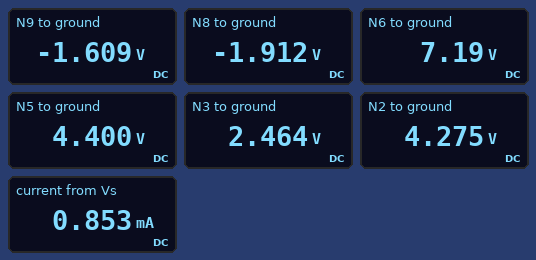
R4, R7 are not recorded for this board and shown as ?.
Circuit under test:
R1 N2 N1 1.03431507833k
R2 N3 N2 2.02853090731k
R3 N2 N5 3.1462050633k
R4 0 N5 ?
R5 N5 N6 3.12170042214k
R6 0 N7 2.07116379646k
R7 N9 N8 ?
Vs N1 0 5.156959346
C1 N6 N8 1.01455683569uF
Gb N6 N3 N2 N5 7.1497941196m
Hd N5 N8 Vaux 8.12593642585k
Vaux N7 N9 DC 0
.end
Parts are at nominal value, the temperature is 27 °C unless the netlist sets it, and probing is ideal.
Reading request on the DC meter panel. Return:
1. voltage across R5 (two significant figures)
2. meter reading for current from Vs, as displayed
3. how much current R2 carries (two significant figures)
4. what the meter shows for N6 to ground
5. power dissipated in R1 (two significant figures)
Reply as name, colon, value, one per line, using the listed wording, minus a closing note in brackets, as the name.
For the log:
voltage across R5: 2.8 V
meter reading for current from Vs, as displayed: 0.853 mA
how much current R2 carries: 890 µA
what the meter shows for N6 to ground: 7.19 V
power dissipated in R1: 750 µW
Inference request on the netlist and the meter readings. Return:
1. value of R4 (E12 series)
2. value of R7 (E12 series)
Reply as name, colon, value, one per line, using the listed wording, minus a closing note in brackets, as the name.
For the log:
value of R4: 2.7 kΩ
value of R7: 390 Ω
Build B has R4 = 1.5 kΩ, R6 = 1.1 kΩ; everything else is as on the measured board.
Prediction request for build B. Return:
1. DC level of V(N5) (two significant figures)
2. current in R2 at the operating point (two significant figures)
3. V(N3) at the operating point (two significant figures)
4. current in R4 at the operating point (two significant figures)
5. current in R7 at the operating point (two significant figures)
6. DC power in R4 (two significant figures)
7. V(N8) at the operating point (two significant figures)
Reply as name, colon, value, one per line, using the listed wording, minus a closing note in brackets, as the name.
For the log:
DC level of V(N5): 3.5 V
current in R2 at the operating point: 1.9 mA
V(N3) at the operating point: -600 mV
current in R4 at the operating point: 2.4 mA
current in R7 at the operating point: 530 µA
DC power in R4: 8.3 mW
V(N8) at the operating point: -790 mV
